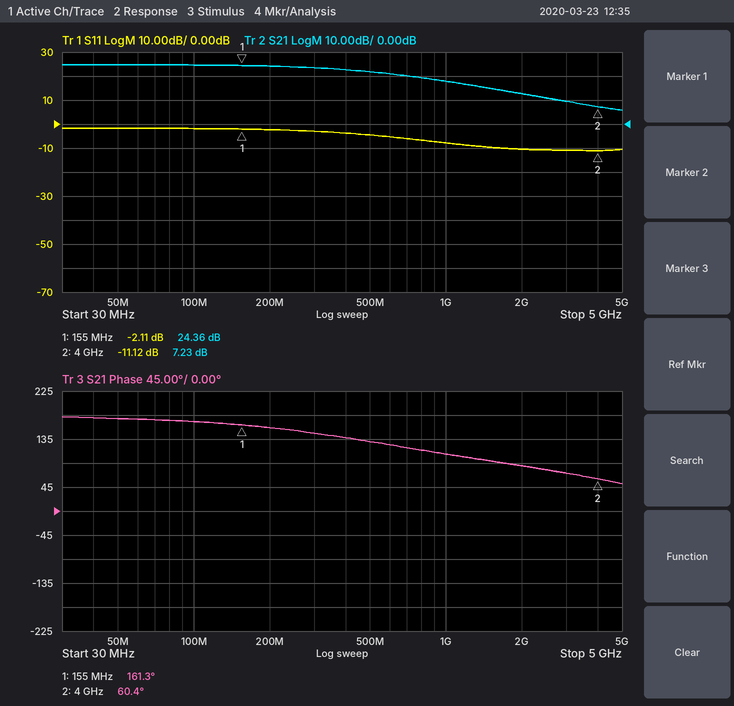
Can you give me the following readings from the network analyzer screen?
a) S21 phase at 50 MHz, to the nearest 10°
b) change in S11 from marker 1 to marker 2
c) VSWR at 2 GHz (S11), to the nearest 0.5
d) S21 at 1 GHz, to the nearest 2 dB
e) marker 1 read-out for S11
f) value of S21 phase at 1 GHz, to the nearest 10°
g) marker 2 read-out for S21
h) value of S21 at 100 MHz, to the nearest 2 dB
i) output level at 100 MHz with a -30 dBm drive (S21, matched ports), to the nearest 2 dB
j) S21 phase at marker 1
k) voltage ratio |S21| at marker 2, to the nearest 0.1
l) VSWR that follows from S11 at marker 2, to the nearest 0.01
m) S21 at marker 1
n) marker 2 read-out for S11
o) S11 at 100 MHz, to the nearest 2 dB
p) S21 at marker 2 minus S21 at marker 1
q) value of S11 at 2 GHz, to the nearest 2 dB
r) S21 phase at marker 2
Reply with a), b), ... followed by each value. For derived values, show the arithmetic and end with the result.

a) 170°
b) -11.12 − (-2.11) = -9.01 dB
c) |Γ| = 10^(-10/20) = 0.3162; VSWR = (1 + 0.3162)/(1 − 0.3162) ≈ 1.92, so 2.0 to the nearest 0.5
d) 18 dB
e) -2.11 dB
f) 110°
g) 7.23 dB
h) 24 dB
i) -30 dBm + (24 dB) = -6 dBm
j) 161.3°
k) 10^(7.23/20) ≈ 2.3
l) (1 + 0.2780)/(1 − 0.2780) ≈ 1.77
m) 24.36 dB
n) -11.12 dB
o) -2 dB
p) 7.23 − (24.36) = -17.13 dB
q) -10 dB
r) 60.4°
